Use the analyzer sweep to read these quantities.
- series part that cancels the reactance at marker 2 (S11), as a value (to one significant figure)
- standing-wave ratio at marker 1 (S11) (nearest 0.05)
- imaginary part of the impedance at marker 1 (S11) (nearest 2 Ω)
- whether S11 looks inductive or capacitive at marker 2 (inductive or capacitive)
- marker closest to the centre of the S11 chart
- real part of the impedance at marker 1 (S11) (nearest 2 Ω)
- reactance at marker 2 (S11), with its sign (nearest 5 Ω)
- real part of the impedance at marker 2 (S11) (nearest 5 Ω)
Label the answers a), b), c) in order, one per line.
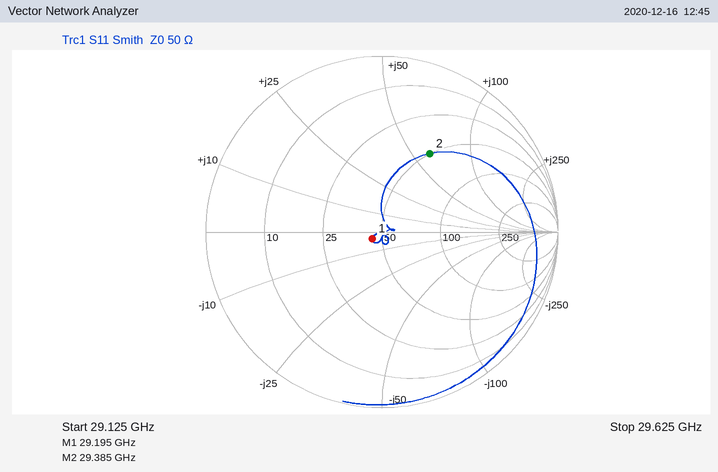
a) 90 fF
b) 1.15
c) -4 Ω
d) inductive
e) marker 1
f) 44 Ω
g) +60 Ω
h) 50 Ω
